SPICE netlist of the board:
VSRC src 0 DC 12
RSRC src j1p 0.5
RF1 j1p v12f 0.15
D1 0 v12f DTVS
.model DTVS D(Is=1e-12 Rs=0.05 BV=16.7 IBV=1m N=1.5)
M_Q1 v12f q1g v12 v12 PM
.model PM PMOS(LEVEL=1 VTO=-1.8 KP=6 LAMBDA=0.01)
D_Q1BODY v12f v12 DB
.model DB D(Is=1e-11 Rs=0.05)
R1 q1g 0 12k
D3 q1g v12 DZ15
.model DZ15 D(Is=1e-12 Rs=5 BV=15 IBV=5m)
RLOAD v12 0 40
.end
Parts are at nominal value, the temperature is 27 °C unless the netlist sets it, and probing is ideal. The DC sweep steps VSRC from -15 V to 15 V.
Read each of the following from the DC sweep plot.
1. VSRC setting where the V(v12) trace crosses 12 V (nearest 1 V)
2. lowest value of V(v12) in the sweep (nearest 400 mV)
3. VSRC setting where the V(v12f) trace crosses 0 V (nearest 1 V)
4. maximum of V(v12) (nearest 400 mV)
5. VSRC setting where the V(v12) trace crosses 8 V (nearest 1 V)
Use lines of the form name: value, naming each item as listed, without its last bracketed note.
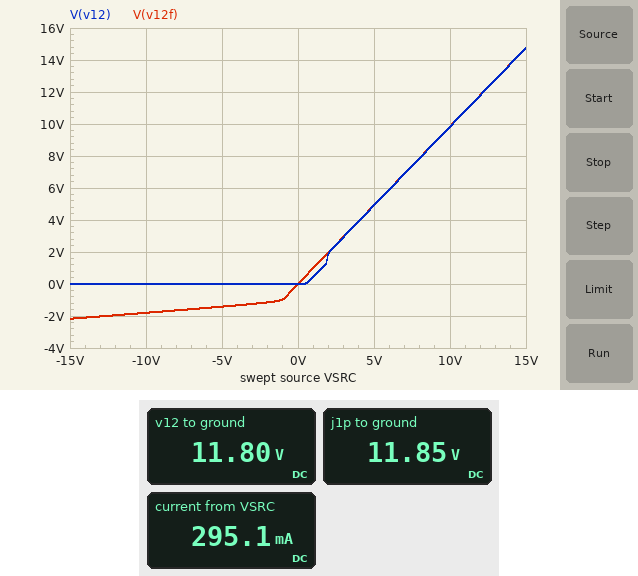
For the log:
VSRC setting where the V(v12) trace crosses 12 V: 12 V
lowest value of V(v12) in the sweep: 0 V
VSRC setting where the V(v12f) trace crosses 0 V: 0 V
maximum of V(v12): 14.8 V
VSRC setting where the V(v12) trace crosses 8 V: 8 V
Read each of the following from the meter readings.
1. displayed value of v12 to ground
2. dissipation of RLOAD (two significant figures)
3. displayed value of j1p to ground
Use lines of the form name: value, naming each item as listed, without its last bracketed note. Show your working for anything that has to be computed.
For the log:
displayed value of v12 to ground: 11.80 V
dissipation of RLOAD: (11.8 V)^2 / 40 Ω = 3.5 W
displayed value of j1p to ground: 11.85 V
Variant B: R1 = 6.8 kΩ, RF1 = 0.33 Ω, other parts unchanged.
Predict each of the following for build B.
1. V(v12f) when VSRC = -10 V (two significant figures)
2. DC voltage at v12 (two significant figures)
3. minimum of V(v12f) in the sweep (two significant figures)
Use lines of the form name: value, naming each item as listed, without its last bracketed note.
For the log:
V(v12f) when VSRC = -10 V: -1.7 V
DC voltage at v12: 12 V
minimum of V(v12f) in the sweep: -2.0 V
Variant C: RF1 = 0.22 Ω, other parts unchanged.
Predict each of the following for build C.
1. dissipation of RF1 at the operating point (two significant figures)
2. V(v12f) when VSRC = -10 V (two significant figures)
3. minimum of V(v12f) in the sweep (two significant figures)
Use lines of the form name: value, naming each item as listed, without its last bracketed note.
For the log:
dissipation of RF1 at the operating point: 19 mW
V(v12f) when VSRC = -10 V: -1.7 V
minimum of V(v12f) in the sweep: -2.1 V
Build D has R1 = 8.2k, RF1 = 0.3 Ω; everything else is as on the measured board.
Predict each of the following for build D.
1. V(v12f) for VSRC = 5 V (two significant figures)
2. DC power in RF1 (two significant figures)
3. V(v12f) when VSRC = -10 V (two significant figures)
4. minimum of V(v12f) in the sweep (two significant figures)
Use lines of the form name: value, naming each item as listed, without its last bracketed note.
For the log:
V(v12f) for VSRC = 5 V: 4.9 V
DC power in RF1: 26 mW
V(v12f) when VSRC = -10 V: -1.7 V
minimum of V(v12f) in the sweep: -2.0 V
